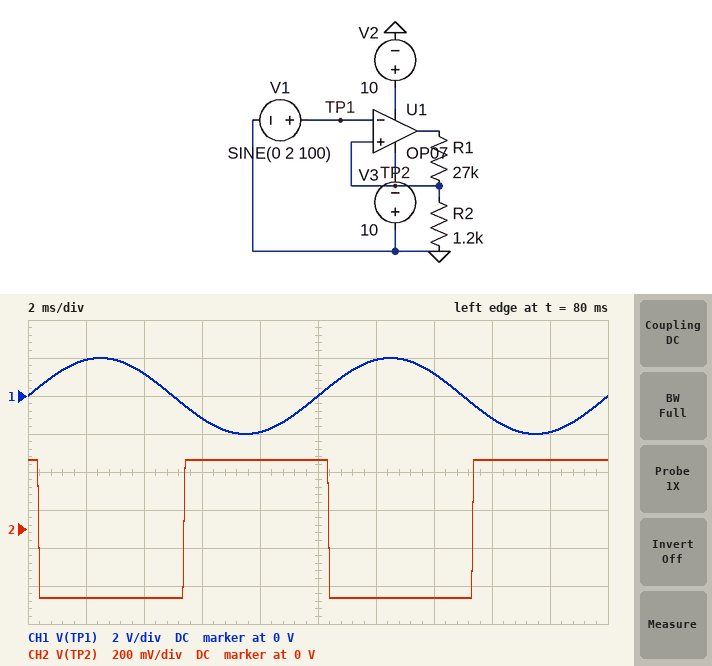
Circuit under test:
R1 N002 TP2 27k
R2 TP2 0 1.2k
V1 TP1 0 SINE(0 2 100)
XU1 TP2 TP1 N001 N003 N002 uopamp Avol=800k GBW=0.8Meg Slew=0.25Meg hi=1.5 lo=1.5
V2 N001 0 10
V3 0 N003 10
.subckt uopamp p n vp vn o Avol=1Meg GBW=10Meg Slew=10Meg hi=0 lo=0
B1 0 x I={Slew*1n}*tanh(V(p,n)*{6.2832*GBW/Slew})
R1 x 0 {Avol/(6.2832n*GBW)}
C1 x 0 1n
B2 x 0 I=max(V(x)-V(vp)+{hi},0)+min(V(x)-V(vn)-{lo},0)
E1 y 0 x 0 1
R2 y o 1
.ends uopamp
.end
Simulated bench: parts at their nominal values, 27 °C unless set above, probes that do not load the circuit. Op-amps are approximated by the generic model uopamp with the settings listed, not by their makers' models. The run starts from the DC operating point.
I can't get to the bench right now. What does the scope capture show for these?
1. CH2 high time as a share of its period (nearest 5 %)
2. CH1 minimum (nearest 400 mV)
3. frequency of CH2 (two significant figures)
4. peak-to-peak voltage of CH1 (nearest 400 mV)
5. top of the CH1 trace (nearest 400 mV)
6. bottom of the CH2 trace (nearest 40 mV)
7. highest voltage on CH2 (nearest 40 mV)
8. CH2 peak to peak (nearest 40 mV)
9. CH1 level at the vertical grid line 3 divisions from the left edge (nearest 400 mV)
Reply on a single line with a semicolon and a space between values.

50 %; -2.0 V; 100 Hz; 4.0 V; 2.0 V; -360 mV; 360 mV; 720 mV; -1.2 V
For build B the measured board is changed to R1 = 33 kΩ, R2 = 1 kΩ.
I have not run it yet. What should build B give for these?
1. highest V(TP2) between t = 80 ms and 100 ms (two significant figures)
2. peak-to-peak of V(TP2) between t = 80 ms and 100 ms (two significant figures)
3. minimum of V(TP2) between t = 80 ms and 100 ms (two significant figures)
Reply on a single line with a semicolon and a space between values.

250 mV; 500 mV; -250 mV
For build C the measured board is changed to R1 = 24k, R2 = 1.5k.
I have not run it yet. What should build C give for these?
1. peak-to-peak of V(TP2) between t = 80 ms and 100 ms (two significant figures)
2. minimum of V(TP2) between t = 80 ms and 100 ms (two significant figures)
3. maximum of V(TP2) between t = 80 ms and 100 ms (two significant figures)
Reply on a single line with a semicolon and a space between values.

1.0 V; -500 mV; 500 mV
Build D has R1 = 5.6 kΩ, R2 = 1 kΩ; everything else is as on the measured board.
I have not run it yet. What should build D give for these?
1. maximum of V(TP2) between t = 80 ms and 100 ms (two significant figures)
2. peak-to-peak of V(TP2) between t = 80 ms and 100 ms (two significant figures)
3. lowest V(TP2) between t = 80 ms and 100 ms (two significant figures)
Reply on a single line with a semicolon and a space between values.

1.3 V; 2.6 V; -1.3 V
